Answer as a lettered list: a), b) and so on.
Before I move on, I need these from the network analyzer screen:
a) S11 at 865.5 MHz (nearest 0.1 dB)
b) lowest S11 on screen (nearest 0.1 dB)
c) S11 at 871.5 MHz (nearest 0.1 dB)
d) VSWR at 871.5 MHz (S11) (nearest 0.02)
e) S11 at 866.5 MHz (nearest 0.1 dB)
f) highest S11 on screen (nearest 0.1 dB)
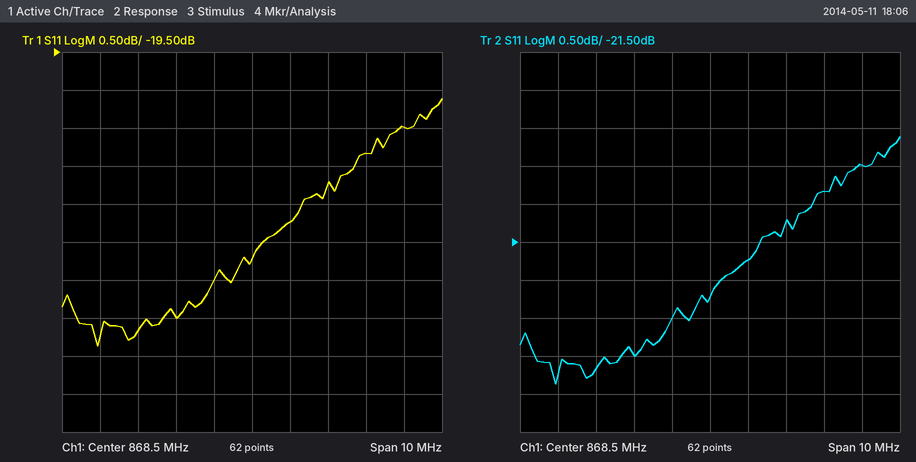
a) -23.2 dB
b) -23.4 dB
c) -20.8 dB
d) 1.20
e) -23.0 dB
f) -20.1 dB
